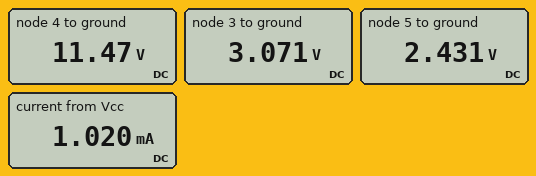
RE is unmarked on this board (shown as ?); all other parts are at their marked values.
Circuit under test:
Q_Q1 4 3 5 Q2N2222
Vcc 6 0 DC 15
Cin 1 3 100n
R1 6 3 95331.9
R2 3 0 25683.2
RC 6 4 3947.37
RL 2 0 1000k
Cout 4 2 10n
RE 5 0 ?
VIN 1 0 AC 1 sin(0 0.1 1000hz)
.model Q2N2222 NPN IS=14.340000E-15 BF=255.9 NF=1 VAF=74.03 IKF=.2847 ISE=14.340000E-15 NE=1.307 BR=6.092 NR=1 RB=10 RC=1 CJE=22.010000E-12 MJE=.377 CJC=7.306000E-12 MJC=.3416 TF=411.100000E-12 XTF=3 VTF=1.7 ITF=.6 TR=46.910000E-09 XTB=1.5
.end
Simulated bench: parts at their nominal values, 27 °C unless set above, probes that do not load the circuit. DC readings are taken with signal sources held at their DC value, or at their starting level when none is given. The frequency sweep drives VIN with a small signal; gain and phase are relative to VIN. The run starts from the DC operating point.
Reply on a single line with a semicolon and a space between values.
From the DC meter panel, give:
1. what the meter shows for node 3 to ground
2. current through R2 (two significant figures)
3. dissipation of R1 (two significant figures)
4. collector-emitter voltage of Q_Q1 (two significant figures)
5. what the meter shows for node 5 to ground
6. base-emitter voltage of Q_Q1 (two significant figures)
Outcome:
3.071 V; 120 µA; 1.5 mW; 9.0 V; 2.431 V; 640 mV
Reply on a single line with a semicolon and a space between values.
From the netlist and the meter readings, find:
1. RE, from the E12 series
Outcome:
2.7 kΩ
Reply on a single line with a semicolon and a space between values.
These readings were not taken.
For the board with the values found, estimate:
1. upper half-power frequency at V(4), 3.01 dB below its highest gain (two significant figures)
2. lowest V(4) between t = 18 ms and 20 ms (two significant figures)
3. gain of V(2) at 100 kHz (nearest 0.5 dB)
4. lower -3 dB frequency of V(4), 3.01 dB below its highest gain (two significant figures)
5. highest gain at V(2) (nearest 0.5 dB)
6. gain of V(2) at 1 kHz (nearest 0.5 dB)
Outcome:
310 MHz; 11 V; 3.0 dB; 82 Hz; 3.0 dB; 3.0 dB
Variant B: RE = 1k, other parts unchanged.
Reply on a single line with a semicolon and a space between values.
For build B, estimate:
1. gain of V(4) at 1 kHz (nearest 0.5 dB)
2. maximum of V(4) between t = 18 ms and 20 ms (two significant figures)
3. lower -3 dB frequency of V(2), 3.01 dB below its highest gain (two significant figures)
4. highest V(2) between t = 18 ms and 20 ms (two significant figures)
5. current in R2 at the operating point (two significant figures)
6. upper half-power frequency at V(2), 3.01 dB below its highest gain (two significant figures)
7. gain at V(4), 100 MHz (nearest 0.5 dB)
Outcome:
11.5 dB; 6.6 V; 91 Hz; 380 mV; 110 µA; 11 MHz; 1.5 dB
